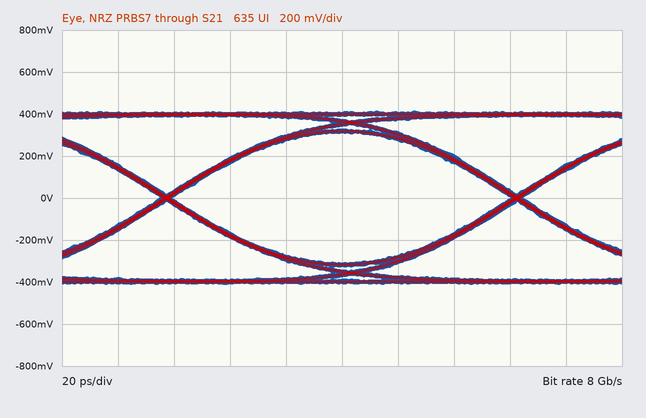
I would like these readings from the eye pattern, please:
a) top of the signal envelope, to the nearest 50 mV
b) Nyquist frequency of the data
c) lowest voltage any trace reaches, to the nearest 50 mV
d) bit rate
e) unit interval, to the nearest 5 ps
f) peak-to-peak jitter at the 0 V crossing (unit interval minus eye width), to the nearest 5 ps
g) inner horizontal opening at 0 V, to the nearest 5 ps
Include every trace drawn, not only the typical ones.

400 mV
4 GHz
-400 mV
8 Gb/s
125 ps
5 ps
120 ps
